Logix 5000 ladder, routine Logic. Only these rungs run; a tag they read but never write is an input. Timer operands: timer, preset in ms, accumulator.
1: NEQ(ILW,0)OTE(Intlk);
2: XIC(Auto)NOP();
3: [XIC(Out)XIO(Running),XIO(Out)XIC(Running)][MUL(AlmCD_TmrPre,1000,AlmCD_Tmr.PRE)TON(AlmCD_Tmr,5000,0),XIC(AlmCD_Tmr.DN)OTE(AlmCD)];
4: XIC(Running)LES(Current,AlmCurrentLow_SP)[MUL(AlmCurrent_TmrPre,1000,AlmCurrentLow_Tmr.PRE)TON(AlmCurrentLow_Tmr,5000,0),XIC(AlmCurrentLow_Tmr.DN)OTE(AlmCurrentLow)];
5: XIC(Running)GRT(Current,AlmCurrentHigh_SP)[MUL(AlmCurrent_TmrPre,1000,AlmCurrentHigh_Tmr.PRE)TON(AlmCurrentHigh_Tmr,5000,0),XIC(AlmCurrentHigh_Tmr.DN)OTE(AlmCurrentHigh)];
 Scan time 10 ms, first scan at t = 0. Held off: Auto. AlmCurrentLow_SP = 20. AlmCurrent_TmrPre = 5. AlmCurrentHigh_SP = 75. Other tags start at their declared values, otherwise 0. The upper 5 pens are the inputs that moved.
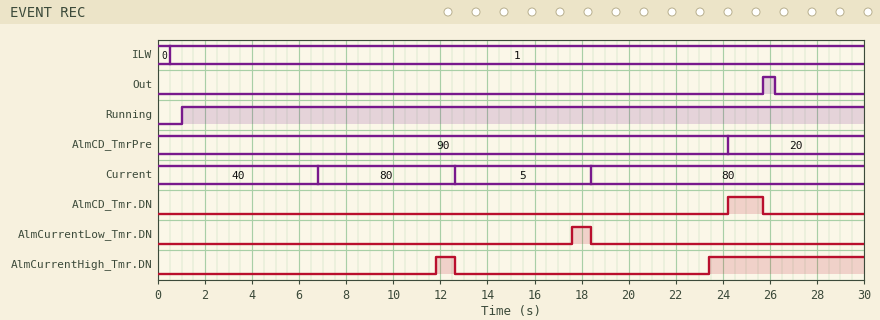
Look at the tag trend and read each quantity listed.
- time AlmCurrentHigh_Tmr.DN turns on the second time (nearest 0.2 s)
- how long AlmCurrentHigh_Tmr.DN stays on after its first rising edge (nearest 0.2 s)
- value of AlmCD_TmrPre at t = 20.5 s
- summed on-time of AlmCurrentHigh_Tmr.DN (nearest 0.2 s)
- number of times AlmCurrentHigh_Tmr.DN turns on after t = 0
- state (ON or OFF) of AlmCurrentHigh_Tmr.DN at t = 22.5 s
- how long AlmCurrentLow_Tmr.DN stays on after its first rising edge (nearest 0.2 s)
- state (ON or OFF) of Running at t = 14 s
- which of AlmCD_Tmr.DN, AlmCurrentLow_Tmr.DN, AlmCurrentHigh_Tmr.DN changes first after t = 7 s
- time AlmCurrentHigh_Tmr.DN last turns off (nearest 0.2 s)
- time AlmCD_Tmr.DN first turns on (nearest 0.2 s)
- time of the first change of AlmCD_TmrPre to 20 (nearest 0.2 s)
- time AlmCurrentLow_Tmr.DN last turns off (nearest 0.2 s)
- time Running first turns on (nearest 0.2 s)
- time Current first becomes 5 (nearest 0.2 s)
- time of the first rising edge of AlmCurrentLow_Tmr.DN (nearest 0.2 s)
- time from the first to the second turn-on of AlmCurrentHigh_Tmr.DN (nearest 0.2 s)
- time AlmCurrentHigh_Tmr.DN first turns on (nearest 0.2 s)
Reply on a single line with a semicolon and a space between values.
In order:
23.4 s; 0.8 s; 90; 7.4 s; 2; OFF; 0.8 s; ON; AlmCurrentHigh_Tmr.DN; 12.6 s; 24.2 s; 24.2 s; 18.4 s; 1.0 s; 12.6 s; 17.6 s; 11.6 s; 11.8 s
